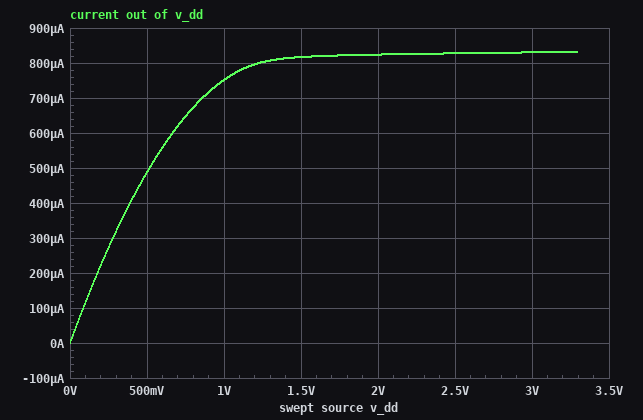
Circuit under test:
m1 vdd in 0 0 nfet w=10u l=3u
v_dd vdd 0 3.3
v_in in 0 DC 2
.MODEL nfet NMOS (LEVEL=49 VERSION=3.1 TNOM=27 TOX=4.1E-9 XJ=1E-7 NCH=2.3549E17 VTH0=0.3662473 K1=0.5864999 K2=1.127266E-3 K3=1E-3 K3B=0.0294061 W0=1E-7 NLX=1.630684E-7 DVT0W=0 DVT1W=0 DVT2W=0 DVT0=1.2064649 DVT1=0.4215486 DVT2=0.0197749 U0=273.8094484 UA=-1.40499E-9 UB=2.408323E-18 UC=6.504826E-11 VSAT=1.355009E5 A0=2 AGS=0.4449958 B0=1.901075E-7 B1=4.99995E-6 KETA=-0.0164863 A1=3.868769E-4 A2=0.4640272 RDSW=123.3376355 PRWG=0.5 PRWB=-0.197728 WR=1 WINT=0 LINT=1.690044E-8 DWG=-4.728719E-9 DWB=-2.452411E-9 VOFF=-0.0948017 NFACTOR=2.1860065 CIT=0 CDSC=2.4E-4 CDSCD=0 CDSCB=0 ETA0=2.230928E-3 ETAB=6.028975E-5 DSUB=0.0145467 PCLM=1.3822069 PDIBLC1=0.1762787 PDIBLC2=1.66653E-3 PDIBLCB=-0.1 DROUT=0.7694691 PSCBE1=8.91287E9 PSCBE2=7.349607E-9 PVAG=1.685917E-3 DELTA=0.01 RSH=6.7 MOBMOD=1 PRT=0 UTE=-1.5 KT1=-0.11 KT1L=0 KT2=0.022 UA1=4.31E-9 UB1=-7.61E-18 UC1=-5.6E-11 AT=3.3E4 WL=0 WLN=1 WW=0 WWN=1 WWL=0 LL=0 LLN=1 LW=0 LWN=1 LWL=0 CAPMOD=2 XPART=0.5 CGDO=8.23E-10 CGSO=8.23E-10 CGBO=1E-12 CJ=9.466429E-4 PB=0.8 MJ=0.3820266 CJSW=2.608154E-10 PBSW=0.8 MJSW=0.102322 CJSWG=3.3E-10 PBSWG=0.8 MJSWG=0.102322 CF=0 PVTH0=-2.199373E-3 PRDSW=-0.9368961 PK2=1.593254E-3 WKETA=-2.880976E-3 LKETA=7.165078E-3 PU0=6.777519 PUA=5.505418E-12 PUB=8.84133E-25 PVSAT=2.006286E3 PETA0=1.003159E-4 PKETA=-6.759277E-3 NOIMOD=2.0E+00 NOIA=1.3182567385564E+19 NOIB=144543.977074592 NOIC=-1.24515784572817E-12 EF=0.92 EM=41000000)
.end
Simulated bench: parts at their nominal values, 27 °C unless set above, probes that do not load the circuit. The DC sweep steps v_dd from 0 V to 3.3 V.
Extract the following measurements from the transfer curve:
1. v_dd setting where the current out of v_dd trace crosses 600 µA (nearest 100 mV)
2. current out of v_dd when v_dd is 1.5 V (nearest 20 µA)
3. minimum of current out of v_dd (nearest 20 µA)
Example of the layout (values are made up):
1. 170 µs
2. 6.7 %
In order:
1. 700 mV
2. 820 µA
3. 0 A
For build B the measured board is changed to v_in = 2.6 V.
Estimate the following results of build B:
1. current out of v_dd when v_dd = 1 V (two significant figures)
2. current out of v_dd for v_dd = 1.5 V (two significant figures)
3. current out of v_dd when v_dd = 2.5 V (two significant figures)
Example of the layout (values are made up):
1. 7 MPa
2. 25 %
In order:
1. 980 µA
2. 1.2 mA
3. 1.4 mA
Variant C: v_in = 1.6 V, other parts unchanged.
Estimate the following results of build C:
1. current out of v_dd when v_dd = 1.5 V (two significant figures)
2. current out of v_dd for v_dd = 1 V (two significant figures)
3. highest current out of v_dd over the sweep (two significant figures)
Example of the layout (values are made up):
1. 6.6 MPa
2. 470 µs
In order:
1. 500 µA
2. 490 µA
3. 510 µA
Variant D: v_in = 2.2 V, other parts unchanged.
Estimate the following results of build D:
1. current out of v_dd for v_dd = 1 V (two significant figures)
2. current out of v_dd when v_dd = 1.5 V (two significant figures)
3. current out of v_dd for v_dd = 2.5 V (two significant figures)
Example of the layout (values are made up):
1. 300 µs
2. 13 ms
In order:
1. 850 µA
2. 980 µA
3. 1.0 mA
